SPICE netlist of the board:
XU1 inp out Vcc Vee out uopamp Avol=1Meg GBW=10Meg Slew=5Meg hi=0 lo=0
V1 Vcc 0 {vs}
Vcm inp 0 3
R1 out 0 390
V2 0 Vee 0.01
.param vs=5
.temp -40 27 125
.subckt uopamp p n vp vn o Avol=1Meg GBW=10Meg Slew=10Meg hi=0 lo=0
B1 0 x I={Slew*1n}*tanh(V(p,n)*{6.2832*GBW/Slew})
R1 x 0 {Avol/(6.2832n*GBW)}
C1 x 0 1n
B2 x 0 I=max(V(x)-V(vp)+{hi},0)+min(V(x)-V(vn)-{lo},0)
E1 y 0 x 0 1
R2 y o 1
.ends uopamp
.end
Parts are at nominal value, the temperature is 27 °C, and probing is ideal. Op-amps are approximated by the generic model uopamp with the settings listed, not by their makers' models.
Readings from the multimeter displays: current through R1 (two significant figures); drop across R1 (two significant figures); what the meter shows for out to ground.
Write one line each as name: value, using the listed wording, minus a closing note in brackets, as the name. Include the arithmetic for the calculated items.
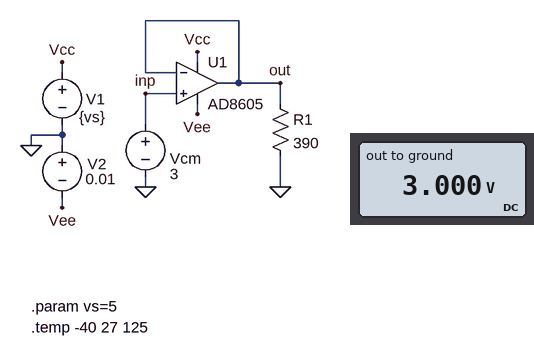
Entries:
current through R1: (3 V) / 390 Ω = 7.7 mA
drop across R1: 3 V = 3.0 V
what the meter shows for out to ground: 3.000 V
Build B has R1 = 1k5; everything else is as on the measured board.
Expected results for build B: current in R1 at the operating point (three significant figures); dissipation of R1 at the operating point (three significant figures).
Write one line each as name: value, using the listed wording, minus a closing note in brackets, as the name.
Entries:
current in R1 at the operating point: 2.00 mA
dissipation of R1 at the operating point: 6.00 mW
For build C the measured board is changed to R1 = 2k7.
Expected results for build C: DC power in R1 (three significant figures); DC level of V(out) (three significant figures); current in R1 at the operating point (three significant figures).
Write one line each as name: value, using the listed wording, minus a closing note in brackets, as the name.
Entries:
DC power in R1: 3.33 mW
DC level of V(out): 3.00 V
current in R1 at the operating point: 1.11 mA
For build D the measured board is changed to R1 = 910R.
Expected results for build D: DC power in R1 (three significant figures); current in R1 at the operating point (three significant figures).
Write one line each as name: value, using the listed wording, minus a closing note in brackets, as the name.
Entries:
DC power in R1: 9.89 mW
current in R1 at the operating point: 3.30 mA
